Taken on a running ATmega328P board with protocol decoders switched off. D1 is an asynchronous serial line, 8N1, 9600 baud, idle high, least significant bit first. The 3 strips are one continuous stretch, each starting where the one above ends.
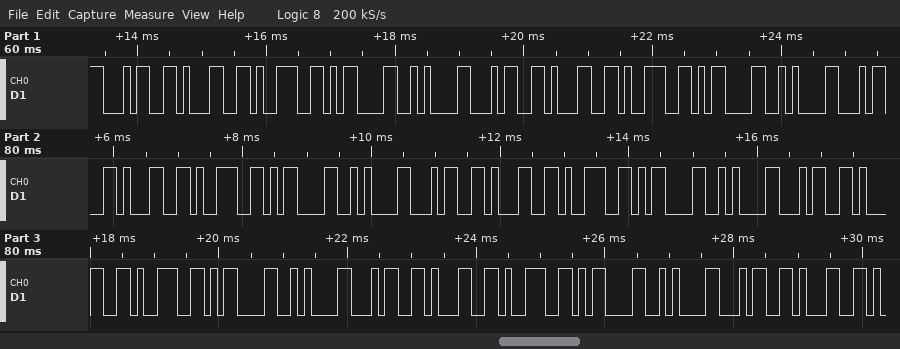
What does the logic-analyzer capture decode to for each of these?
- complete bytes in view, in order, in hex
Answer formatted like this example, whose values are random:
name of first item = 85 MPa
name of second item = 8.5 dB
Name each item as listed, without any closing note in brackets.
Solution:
complete bytes in view, in order, in hex = 34 31 39 0D 0A 34 31 39 0D 0A 34 31 39 0D 0A 34 31 39 0D 0A 34 31 39 0D 0A 34 31 39 0D 0A 34 31
